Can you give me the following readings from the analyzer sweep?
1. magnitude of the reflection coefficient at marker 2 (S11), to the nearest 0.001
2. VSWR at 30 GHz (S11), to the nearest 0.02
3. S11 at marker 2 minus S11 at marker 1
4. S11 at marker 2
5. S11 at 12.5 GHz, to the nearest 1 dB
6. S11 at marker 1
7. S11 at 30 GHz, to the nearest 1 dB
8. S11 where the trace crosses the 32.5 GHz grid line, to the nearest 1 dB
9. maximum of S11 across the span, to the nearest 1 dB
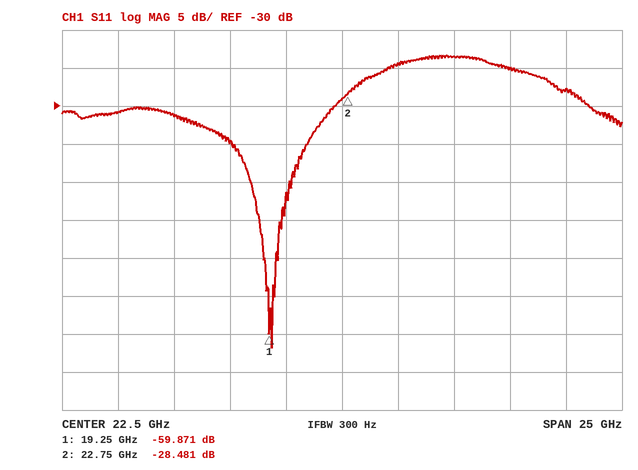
0.038
1.12
31.390 dB
-28.481 dB
-31 dB
-59.871 dB
-25 dB
-28 dB
-23 dB
